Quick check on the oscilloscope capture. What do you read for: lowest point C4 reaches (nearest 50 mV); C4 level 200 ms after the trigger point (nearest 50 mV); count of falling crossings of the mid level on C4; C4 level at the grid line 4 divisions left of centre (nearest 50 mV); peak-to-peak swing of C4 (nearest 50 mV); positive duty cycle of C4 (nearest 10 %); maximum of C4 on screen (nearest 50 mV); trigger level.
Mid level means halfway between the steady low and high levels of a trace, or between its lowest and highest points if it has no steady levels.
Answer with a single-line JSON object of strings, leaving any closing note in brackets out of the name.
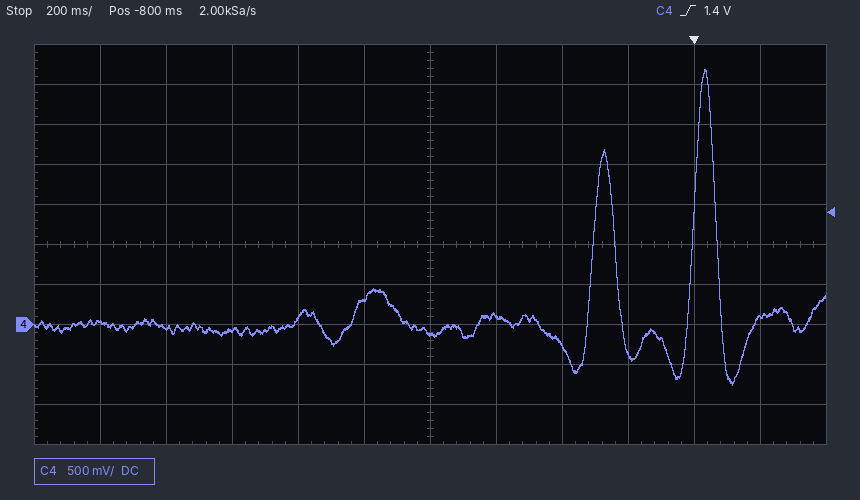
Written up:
{"lowest point C4 reaches": "-750 mV", "C4 level 200 ms after the trigger point": "100 mV", "count of falling crossings of the mid level on C4": "2", "C4 level at the grid line 4 divisions left of centre": "-50 mV", "peak-to-peak swing of C4": "3.95 V", "positive duty cycle of C4": "20 %", "maximum of C4 on screen": "3.20 V", "trigger level": "1.4 V"}
